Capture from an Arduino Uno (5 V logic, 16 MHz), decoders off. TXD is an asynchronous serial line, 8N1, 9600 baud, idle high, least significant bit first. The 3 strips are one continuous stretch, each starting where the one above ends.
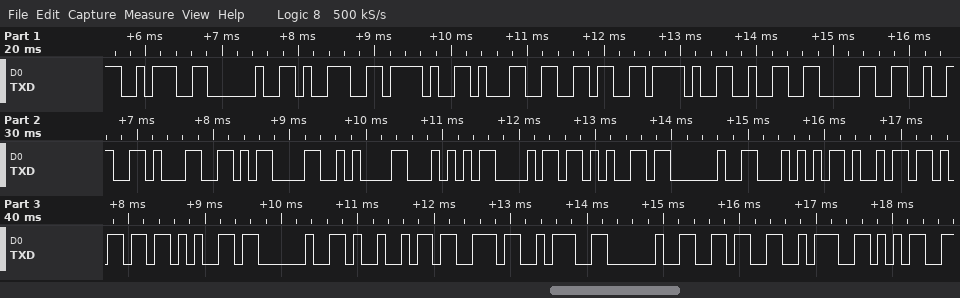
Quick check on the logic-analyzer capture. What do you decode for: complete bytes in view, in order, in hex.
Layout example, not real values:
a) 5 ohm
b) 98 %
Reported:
a) 0x3A 0x20 0x39 0x2F 0x31 0x36 0x2F 0x32 0x30 0x32 0x31 0x0D 0x0A 0x54 0x68 0x65 0x20 0x54 0x69 0x6D 0x65 0x20 0x49 0x73 0x3A 0x20 0x36 0x3A 0x35
